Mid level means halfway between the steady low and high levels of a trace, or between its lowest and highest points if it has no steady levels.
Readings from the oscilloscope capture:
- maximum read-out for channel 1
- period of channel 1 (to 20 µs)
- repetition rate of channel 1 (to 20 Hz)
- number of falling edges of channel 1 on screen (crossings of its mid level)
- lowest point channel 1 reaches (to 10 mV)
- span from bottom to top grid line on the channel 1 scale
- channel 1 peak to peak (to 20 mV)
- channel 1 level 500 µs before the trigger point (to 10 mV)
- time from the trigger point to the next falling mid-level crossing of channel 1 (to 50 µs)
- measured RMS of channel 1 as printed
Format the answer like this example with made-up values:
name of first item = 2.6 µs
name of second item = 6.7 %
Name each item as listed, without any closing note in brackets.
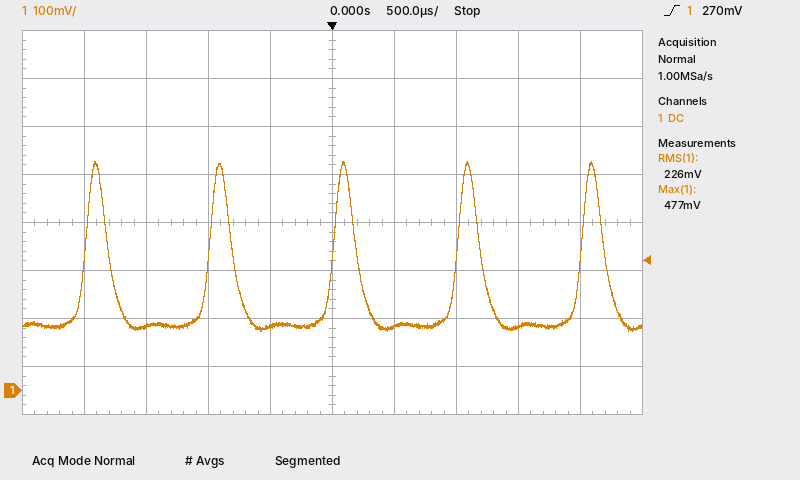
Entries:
maximum read-out for channel 1 = 477 mV
period of channel 1 = 1.00 ms
repetition rate of channel 1 = 1.00 kHz
number of falling edges of channel 1 on screen = 5
lowest point channel 1 reaches = 120 mV
span from bottom to top grid line on the channel 1 scale = 800 mV
channel 1 peak to peak = 360 mV
channel 1 level 500 µs before the trigger point = 130 mV
time from the trigger point to the next falling mid-level crossing of channel 1 = 200 µs
measured RMS of channel 1 as printed = 226 mV
